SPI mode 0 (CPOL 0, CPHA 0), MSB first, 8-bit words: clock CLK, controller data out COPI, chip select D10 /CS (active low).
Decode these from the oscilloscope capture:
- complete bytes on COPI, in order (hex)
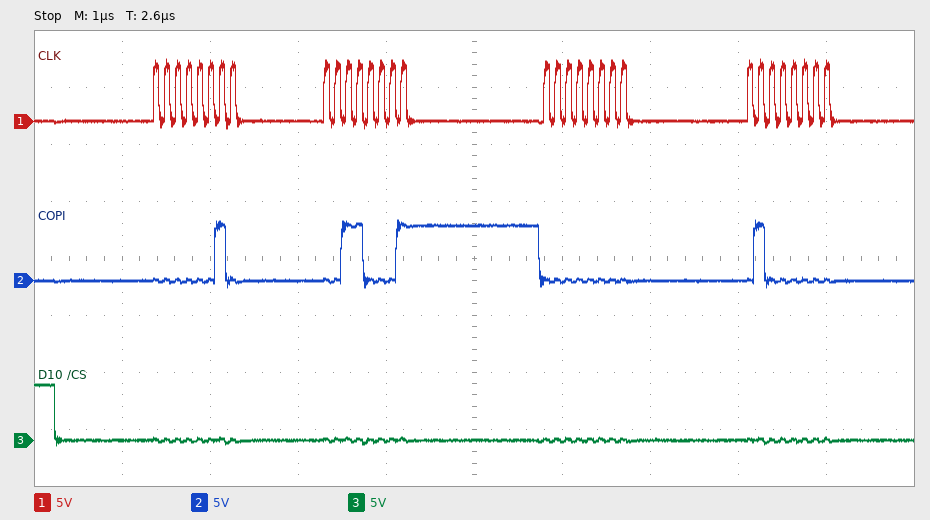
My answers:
02 31 00 40
